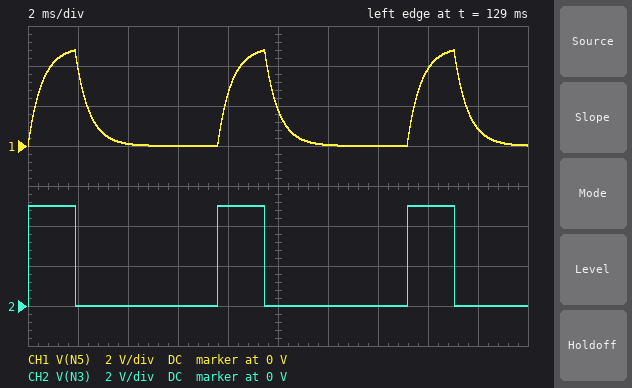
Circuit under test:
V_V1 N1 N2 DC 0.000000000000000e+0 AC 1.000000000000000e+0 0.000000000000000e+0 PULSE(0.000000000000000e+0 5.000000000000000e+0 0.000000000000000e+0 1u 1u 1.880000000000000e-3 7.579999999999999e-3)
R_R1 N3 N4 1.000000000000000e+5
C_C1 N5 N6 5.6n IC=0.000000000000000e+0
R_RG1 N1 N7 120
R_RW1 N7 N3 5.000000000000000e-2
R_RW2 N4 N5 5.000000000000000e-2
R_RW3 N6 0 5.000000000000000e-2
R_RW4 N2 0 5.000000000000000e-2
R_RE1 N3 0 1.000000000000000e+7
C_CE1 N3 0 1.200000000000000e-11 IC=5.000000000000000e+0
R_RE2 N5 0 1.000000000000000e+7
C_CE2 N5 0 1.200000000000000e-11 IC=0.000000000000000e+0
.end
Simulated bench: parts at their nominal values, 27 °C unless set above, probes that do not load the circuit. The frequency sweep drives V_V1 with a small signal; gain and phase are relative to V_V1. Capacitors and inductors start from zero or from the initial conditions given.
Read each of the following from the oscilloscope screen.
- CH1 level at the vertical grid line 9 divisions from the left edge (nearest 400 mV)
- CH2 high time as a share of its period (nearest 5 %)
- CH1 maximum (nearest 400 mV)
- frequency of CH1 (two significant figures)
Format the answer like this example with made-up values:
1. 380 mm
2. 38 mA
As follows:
1. 800 mV
2. 25 %
3. 4.8 V
4. 130 Hz
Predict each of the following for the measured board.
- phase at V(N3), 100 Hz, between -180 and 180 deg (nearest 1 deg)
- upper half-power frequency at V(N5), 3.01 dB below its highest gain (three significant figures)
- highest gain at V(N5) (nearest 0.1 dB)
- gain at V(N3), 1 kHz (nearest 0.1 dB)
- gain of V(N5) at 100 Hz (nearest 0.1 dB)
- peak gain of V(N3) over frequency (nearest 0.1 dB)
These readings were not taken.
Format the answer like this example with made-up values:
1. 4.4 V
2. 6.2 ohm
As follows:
1. 0 deg
2. 286 Hz
3. -0.1 dB
4. 0 dB
5. -0.6 dB
6. 0 dB
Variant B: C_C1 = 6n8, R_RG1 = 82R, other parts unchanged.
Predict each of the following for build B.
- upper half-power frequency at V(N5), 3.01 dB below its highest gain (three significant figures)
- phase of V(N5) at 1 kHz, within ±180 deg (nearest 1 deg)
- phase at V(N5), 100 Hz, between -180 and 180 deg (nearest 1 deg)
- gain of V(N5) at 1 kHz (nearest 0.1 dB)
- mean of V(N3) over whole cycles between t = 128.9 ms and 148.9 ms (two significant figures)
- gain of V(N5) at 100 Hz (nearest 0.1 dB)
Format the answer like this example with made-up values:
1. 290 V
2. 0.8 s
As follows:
1. 236 Hz
2. -77 deg
3. -23 deg
4. -12.9 dB
5. 1.2 V
6. -0.8 dB
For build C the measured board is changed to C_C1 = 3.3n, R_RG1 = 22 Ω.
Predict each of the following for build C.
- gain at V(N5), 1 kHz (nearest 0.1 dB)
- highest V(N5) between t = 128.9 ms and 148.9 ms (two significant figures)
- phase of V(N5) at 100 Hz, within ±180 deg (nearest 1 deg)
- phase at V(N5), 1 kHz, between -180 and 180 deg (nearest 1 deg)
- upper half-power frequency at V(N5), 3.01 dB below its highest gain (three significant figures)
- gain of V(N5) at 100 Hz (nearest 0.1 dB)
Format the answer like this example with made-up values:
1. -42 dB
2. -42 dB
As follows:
1. -7.3 dB
2. 4.9 V
3. -12 deg
4. -64 deg
5. 485 Hz
6. -0.3 dB
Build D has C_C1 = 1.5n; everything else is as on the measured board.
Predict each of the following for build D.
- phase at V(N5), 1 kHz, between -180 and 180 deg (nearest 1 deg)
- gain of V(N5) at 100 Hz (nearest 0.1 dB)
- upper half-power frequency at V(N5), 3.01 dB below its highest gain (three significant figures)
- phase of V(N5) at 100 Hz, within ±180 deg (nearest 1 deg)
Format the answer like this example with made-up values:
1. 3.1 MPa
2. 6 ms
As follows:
1. -43 deg
2. -0.1 dB
3. 1.06 kHz
4. -5 deg
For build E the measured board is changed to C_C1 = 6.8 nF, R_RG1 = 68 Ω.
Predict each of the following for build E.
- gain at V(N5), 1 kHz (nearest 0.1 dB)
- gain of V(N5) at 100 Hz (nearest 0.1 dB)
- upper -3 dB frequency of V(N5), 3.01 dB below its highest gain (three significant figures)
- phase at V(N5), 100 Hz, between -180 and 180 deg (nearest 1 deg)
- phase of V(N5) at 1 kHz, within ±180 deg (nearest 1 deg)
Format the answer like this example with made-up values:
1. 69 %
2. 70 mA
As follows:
1. -12.9 dB
2. -0.8 dB
3. 236 Hz
4. -23 deg
5. -77 deg
